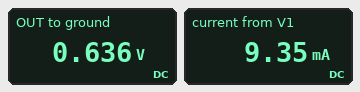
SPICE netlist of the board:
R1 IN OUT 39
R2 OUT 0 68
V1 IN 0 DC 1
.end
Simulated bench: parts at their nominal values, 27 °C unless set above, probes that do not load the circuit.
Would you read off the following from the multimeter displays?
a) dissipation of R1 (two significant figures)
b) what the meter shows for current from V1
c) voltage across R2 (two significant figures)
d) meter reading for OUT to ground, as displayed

3.4 mW
9.35 mA
640 mV
0.636 V
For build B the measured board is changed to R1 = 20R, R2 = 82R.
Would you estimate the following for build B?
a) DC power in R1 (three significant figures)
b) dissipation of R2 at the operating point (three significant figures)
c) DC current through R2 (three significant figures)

1.92 mW
7.88 mW
9.80 mA
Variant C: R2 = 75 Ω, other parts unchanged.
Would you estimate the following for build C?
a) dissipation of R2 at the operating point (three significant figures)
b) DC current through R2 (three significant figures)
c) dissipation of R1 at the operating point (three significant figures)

5.77 mW
8.77 mA
3.00 mW
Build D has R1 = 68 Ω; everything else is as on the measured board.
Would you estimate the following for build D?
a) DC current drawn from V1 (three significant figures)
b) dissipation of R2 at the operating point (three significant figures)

7.35 mA
3.68 mW
